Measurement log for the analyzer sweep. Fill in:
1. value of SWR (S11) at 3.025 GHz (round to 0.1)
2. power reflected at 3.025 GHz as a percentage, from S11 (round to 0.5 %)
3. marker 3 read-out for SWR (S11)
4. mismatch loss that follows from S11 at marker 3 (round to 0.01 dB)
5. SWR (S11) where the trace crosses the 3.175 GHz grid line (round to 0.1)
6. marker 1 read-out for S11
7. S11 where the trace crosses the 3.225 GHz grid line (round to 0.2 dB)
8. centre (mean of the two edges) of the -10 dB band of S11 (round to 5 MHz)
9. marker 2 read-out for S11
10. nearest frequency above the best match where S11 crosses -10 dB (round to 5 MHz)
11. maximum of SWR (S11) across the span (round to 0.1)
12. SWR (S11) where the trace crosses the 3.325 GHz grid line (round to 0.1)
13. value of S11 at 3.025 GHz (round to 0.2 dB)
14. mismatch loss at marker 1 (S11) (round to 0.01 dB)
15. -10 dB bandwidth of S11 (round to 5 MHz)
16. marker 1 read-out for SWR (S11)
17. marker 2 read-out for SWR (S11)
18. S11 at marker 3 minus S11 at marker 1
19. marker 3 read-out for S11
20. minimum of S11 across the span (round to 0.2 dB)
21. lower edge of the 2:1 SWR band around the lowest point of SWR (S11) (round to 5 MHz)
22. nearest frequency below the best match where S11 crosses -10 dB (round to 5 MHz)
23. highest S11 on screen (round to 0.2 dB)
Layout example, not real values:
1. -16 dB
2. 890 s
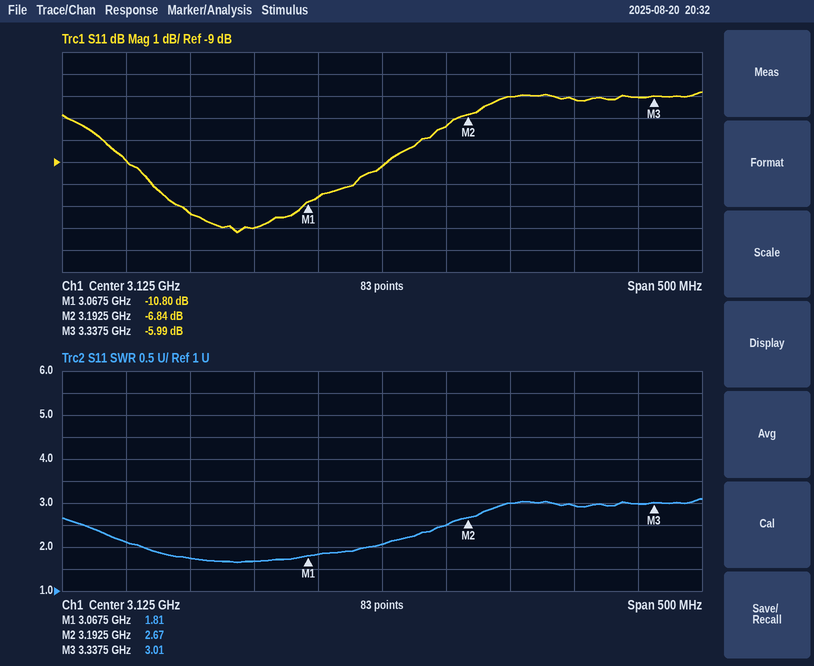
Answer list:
1. 1.7
2. 6.5 %
3. 3.01
4. 1.26 dB
5. 2.5
6. -10.80 dB
7. -6.0 dB
8. 3.025 GHz
9. -6.84 dB
10. 3.105 GHz
11. 3.1
12. 3.0
13. -12.0 dB
14. 0.38 dB
15. 160 MHz
16. 1.81
17. 2.67
18. 4.81 dB
19. -5.99 dB
20. -12.2 dB
21. 2.940 GHz
22. 2.945 GHz
23. -5.8 dB
